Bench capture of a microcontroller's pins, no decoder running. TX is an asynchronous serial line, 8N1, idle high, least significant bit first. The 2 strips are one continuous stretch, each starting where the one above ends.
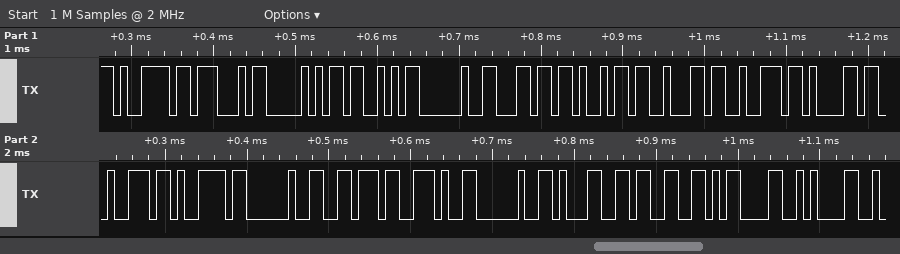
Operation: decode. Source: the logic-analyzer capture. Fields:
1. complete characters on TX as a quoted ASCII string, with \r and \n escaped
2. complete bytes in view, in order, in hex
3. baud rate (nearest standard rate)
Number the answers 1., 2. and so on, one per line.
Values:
1. "yGPS library v. 13\r\n"
2. 0x79 0x47 0x50 0x53 0x20 0x6C 0x69 0x62 0x72 0x61 0x72 0x79 0x20 0x76 0x2E 0x20 0x31 0x33 0x0D 0x0A
3. 115200 baud
